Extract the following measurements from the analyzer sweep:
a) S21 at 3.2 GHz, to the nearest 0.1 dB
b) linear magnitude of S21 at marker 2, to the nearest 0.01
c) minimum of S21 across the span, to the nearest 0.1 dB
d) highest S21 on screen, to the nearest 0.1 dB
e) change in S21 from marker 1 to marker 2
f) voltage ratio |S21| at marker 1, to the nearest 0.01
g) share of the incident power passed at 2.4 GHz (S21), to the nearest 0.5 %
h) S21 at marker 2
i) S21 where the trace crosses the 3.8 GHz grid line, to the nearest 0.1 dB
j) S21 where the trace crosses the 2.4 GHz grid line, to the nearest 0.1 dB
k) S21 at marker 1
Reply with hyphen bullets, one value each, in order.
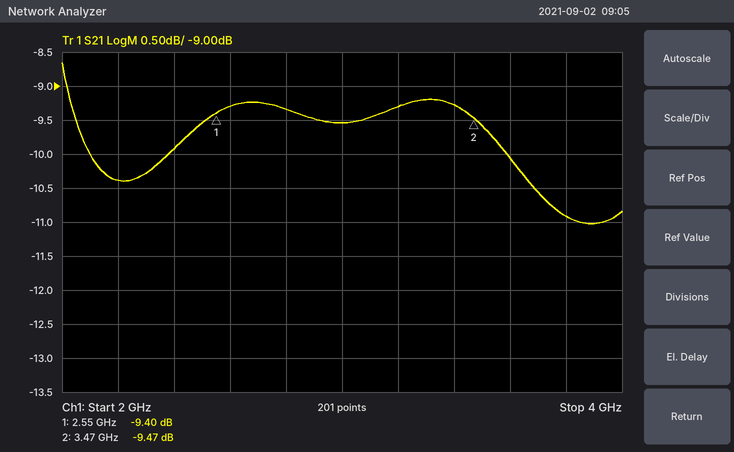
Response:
- -9.3 dB
- 0.34
- -11.0 dB
- -8.7 dB
- -0.07 dB
- 0.34
- 10.0 %
- -9.47 dB
- -10.9 dB
- -9.9 dB
- -9.40 dB
